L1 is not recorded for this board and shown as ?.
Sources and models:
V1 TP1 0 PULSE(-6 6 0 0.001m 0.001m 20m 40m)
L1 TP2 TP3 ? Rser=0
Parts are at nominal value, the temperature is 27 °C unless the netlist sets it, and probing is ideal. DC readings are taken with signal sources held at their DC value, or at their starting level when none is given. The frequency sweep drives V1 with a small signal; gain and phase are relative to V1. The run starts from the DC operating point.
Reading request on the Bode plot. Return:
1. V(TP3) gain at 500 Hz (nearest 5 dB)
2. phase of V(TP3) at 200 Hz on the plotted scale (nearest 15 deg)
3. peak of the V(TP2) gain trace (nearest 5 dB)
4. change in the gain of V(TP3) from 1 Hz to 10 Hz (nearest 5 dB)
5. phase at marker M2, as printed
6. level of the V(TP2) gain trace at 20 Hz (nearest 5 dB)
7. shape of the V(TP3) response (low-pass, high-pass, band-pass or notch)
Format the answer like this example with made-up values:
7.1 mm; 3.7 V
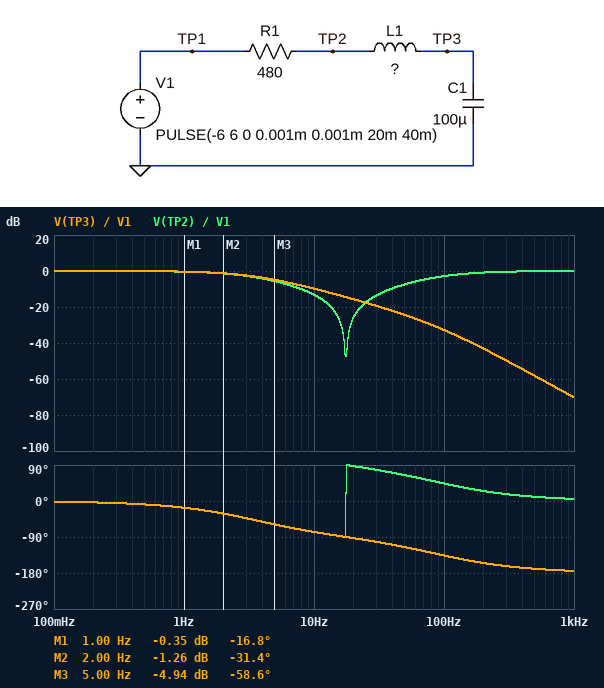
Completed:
-60 dB; -150 deg; 0 dB; -10 dB; -31.4 deg; -25 dB; low-pass
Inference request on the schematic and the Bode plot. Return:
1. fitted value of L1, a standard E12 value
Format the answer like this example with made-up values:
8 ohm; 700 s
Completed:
820 mH
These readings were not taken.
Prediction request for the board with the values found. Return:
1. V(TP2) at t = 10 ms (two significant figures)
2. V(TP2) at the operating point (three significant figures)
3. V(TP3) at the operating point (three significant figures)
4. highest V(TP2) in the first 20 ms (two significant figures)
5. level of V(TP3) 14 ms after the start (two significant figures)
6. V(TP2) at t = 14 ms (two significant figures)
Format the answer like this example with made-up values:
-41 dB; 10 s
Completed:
-4.4 V; -6.00 V; -6.00 V; 6.0 V; -3.2 V; -3.6 V
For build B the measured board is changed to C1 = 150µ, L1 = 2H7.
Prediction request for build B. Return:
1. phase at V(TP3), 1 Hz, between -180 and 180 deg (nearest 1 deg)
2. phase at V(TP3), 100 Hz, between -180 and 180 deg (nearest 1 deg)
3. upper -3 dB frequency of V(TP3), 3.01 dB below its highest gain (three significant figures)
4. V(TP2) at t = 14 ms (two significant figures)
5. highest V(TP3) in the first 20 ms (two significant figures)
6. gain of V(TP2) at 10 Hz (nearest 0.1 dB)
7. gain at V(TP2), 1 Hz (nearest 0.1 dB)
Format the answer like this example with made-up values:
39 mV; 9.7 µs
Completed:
-25 deg; -164 deg; 2.40 Hz; -4.2 V; -3.7 V; -17.6 dB; -0.8 dB
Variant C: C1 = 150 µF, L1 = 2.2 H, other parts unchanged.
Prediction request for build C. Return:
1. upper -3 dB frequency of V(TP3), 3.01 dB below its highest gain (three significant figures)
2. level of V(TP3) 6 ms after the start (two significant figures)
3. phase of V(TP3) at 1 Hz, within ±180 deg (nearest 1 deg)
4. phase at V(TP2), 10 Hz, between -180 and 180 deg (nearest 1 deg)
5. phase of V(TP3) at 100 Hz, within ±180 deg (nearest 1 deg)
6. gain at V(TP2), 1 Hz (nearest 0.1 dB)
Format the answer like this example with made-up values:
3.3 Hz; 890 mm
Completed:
2.36 Hz; -5.6 V; -25 deg; 86 deg; -161 deg; -0.8 dB
